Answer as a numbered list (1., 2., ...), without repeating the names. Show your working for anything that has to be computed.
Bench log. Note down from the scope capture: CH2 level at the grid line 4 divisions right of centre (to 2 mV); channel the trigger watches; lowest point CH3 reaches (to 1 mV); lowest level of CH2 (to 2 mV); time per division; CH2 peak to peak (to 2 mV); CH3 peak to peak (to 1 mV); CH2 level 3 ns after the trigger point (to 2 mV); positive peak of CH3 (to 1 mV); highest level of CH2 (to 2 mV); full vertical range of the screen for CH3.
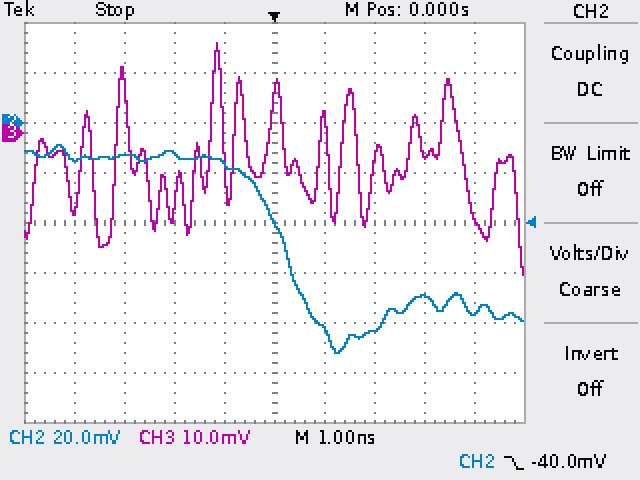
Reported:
1. -76 mV
2. CH2
3. -28 mV
4. -92 mV
5. 1 ns
6. -8 mV − (-92 mV) = 84 mV
7. 18 mV − (-28 mV) = 46 mV
8. -70 mV
9. 18 mV
10. -8 mV
11. 80 mV
